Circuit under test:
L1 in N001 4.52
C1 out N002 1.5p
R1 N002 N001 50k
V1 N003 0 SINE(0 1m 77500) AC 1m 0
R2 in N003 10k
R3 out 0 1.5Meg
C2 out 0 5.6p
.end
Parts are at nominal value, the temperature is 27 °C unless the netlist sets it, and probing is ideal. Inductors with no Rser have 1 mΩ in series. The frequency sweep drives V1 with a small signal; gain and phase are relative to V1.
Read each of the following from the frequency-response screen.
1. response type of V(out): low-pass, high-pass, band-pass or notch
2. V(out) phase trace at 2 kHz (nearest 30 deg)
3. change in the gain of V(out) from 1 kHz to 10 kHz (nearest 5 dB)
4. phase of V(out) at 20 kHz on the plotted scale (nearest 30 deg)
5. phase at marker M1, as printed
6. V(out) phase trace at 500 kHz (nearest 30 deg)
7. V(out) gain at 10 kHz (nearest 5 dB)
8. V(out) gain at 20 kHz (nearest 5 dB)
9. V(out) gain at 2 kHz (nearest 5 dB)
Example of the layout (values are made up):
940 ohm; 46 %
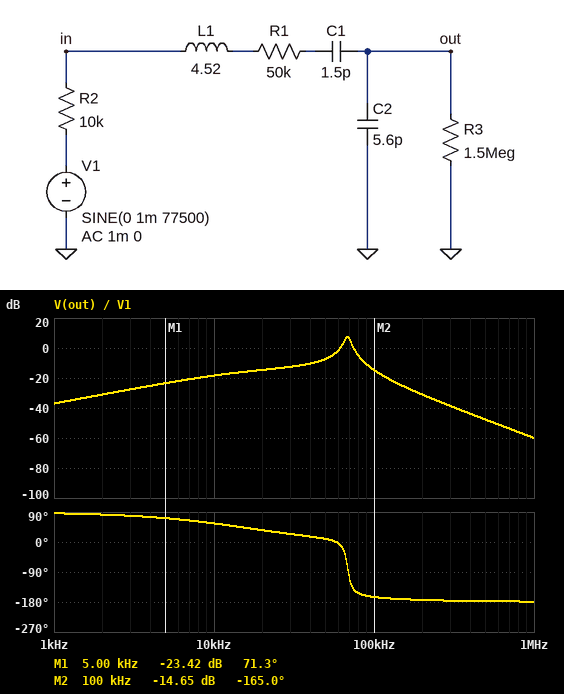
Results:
band-pass; 90 deg; 20 dB; 30 deg; 71.3 deg; -180 deg; -20 dB; -15 dB; -30 dB
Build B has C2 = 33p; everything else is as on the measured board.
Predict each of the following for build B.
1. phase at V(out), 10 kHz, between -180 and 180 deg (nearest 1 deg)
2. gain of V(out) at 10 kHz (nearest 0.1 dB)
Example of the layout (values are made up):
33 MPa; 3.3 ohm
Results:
17 deg; -27.4 dB
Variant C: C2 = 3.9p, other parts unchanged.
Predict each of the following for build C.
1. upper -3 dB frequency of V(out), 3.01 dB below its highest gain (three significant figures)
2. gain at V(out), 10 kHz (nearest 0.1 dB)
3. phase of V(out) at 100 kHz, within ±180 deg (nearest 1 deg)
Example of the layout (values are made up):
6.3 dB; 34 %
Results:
75.2 kHz; -17.8 dB; -158 deg
